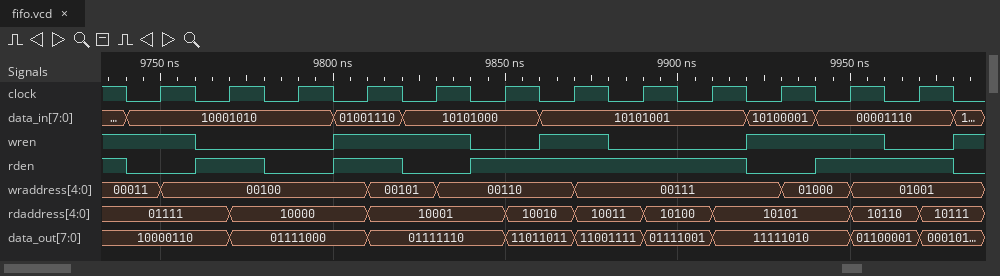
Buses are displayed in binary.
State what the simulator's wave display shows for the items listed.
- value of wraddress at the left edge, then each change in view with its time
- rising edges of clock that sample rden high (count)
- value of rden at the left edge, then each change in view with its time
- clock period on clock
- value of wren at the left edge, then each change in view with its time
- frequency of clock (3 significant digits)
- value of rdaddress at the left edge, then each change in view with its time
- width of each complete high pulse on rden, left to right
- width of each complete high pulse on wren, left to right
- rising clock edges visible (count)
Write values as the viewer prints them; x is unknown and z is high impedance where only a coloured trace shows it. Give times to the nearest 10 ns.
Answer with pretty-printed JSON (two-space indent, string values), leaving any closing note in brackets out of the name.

{
  "value of wraddress at the left edge, then each change in view with its time": "00011, 00100 at 9750 ns, 00101 at 9810 ns, 00110 at 9830 ns, 00111 at 9870 ns, 01000 at 9930 ns, 01001 at 9950 ns",
  "rising edges of clock that sample rden high": "8",
  "value of rden at the left edge, then each change in view with its time": "1, 0 at 9740 ns, 1 at 9760 ns, 0 at 9780 ns, 1 at 9800 ns, 0 at 9820 ns, 1 at 9840 ns, 0 at 9920 ns, 1 at 9940 ns, 0 at 9980 ns",
  "clock period on clock": "20 ns",
  "value of wren at the left edge, then each change in view with its time": "1, 0 at 9760 ns, 1 at 9800 ns, 0 at 9840 ns, 1 at 9860 ns, 0 at 9880 ns, 1 at 9920 ns, 0 at 9960 ns, 1 at 9980 ns",
  "frequency of clock": "50.0 MHz",
  "value of rdaddress at the left edge, then each change in view with its time": "01111, 10000 at 9770 ns, 10001 at 9810 ns, 10010 at 9850 ns, 10011 at 9870 ns, 10100 at 9890 ns, 10101 at 9910 ns, 10110 at 9950 ns, 10111 at 9970 ns",
  "width of each complete high pulse on rden, left to right": "20 ns, 20 ns, 80 ns, 40 ns",
  "width of each complete high pulse on wren, left to right": "40 ns, 20 ns, 40 ns",
  "rising clock edges visible": "12"
}
